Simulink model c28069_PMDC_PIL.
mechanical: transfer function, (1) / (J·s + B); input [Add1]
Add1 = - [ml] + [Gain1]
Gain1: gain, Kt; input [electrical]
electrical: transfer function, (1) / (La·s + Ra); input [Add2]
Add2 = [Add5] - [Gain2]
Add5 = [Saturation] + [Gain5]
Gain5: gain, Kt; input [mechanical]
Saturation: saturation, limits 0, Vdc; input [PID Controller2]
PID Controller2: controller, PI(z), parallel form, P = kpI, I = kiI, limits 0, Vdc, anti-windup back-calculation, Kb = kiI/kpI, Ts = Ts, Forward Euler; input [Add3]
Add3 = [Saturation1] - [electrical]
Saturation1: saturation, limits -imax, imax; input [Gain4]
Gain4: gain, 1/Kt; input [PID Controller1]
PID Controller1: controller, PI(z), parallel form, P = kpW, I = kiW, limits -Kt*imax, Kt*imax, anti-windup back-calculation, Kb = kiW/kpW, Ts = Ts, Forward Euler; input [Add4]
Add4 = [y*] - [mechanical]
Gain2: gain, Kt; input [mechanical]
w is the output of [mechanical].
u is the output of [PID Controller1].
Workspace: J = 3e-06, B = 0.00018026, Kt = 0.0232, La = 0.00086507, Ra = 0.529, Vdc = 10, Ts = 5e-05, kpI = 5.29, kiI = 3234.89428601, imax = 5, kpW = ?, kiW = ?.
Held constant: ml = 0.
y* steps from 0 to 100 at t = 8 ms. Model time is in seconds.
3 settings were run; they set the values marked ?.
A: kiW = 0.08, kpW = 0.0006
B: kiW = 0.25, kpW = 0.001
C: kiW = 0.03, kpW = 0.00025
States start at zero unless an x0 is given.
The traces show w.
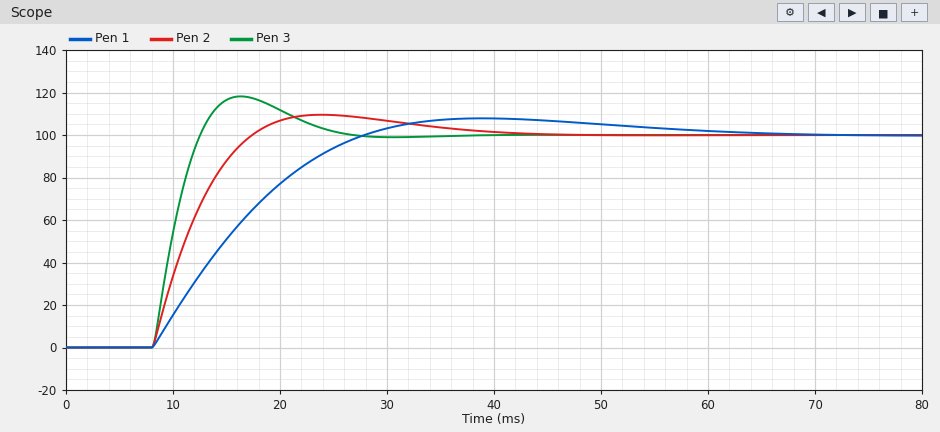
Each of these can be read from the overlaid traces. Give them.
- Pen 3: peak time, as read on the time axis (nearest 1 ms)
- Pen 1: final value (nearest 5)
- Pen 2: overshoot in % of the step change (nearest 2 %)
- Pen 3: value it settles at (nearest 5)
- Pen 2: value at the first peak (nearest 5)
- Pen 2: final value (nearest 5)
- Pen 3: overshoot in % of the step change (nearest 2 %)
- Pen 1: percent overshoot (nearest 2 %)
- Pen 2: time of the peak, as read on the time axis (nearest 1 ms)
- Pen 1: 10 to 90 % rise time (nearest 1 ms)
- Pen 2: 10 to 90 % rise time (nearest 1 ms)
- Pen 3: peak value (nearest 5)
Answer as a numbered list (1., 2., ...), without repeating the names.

1. 16 ms
2. 100
3. 10 %
4. 100
5. 110
6. 100
7. 18 %
8. 8 %
9. 24 ms
10. 14 ms
11. 7 ms
12. 120
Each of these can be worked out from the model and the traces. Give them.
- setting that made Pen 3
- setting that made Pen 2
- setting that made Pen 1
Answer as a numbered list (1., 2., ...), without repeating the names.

1. B
2. A
3. C
